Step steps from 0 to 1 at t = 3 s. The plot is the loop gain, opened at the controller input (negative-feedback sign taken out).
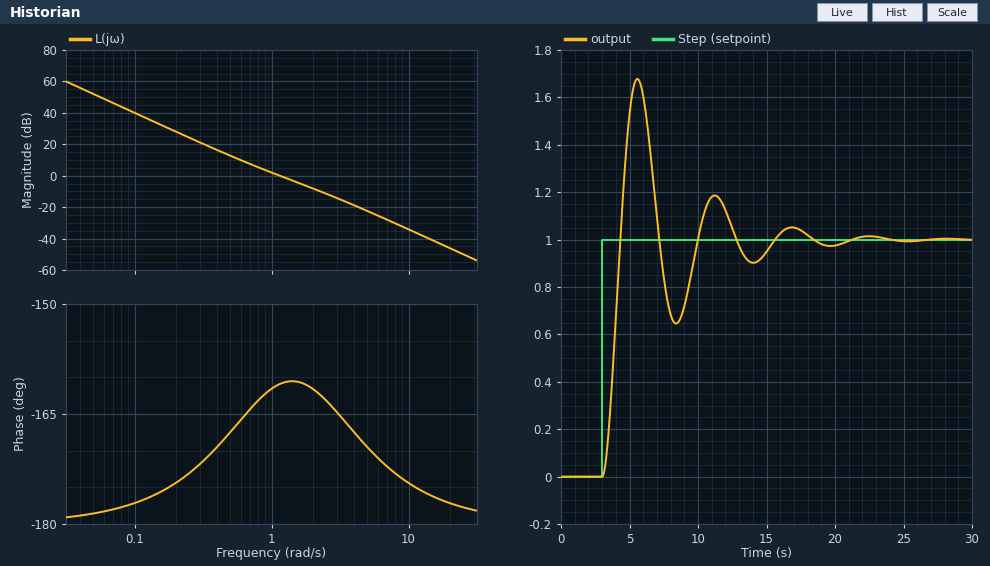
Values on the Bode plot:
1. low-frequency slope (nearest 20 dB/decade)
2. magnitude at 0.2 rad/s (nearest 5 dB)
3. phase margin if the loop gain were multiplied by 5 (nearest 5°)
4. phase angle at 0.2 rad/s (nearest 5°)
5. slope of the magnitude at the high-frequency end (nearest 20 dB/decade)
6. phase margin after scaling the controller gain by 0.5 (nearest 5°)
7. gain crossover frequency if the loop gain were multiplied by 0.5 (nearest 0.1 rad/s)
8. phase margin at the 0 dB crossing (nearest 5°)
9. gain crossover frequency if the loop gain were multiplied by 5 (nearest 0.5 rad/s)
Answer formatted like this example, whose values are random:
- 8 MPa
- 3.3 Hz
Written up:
- -40 dB/decade
- 30 dB
- 15°
- -175°
- -40 dB/decade
- 15°
- 0.8 rad/s
- 20°
- 3.0 rad/s
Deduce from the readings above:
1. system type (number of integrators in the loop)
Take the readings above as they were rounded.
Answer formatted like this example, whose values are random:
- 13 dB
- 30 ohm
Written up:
- 2
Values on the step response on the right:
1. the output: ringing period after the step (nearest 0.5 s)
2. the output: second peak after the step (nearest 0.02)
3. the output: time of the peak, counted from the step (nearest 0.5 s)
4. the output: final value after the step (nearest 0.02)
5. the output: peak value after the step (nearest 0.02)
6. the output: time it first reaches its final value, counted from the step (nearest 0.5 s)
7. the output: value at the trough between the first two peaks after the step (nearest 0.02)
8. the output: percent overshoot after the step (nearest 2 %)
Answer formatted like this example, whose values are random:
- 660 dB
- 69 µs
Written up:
- 5.5 s
- 1.18
- 2.5 s
- 1.00
- 1.68
- 1.5 s
- 0.64
- 68 %
